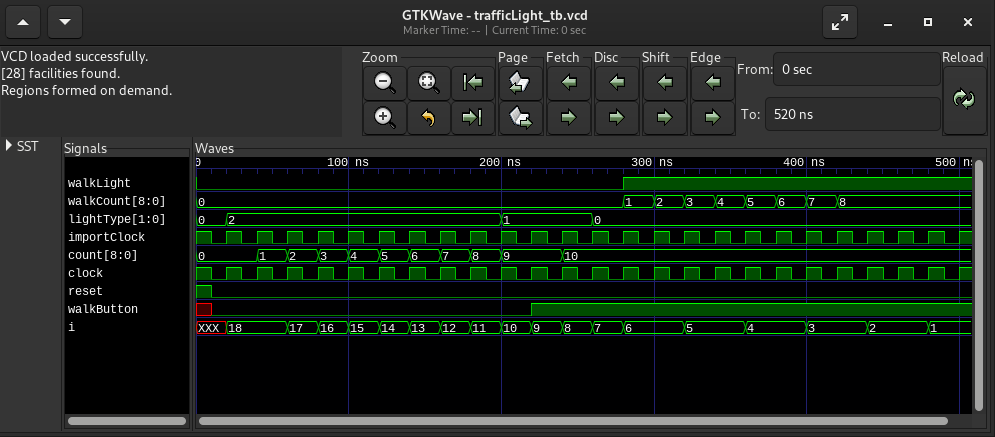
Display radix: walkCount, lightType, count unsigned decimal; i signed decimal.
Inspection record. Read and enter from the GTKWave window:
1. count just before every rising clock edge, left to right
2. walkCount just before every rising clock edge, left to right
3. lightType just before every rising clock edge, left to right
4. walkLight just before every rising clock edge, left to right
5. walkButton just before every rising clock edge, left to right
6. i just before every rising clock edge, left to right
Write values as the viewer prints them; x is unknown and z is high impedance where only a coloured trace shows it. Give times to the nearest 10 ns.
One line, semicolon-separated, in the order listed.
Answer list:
0, 0, 1, 2, 3, 4, 5, 6, 7, 8, 9, 9, 10, 10, 10, 10, 10, 10, 10, 10, 10, 10, 10, 10, 10; 0, 0, 0, 0, 0, 0, 0, 0, 0, 0, 0, 0, 0, 0, 1, 2, 3, 4, 5, 6, 7, 8, 8, 8, 8; 0, 2, 2, 2, 2, 2, 2, 2, 2, 2, 1, 1, 1, 0, 0, 0, 0, 0, 0, 0, 0, 0, 0, 0, 0; 0 0 0 0 0 0 0 0 0 0 0 0 0 0 1 1 1 1 1 1 1 1 1 1 1; 0 0 0 0 0 0 0 0 0 0 0 1 1 1 1 1 1 1 1 1 1 1 1 1 1; XXX, 18, 18, 17, 16, 15, 14, 13, 12, 11, 10, 9, 8, 7, 6, 6, 5, 5, 4, 4, 3, 3, 2, 2, 1
